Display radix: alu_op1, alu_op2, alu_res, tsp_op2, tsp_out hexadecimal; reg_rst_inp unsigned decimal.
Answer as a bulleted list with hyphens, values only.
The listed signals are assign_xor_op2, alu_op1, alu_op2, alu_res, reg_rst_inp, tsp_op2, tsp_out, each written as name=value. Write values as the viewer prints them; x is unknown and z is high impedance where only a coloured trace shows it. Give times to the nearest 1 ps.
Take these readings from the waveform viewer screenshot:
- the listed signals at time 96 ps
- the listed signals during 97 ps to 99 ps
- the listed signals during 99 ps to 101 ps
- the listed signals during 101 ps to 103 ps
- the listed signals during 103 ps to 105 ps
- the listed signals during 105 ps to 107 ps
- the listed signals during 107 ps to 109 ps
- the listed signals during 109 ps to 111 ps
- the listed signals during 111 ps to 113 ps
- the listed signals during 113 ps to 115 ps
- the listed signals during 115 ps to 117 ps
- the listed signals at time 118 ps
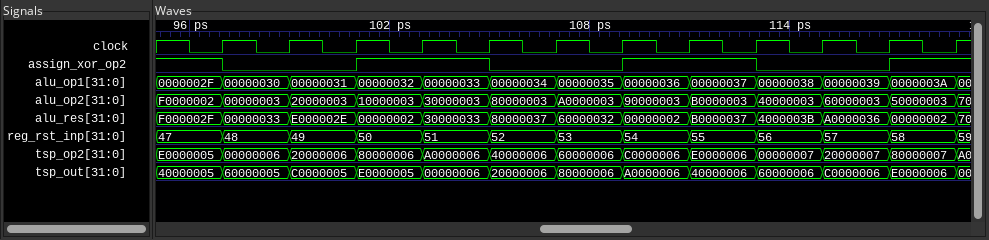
- assign_xor_op2=1, alu_op1=0000002F, alu_op2=F0000002, alu_res=F000002F, reg_rst_inp=47, tsp_op2=E0000005, tsp_out=40000005
- assign_xor_op2=0, alu_op1=00000030, alu_op2=00000003, alu_res=00000033, reg_rst_inp=48, tsp_op2=00000006, tsp_out=60000005
- assign_xor_op2=0, alu_op1=00000031, alu_op2=20000003, alu_res=E000002E, reg_rst_inp=49, tsp_op2=20000006, tsp_out=C0000005
- assign_xor_op2=1, alu_op1=00000032, alu_op2=10000003, alu_res=00000002, reg_rst_inp=50, tsp_op2=80000006, tsp_out=E0000005
- assign_xor_op2=1, alu_op1=00000033, alu_op2=30000003, alu_res=30000033, reg_rst_inp=51, tsp_op2=A0000006, tsp_out=00000006
- assign_xor_op2=0, alu_op1=00000034, alu_op2=80000003, alu_res=80000037, reg_rst_inp=52, tsp_op2=40000006, tsp_out=20000006
- assign_xor_op2=0, alu_op1=00000035, alu_op2=A0000003, alu_res=60000032, reg_rst_inp=53, tsp_op2=60000006, tsp_out=80000006
- assign_xor_op2=1, alu_op1=00000036, alu_op2=90000003, alu_res=00000002, reg_rst_inp=54, tsp_op2=C0000006, tsp_out=A0000006
- assign_xor_op2=1, alu_op1=00000037, alu_op2=B0000003, alu_res=B0000037, reg_rst_inp=55, tsp_op2=E0000006, tsp_out=40000006
- assign_xor_op2=0, alu_op1=00000038, alu_op2=40000003, alu_res=4000003B, reg_rst_inp=56, tsp_op2=00000007, tsp_out=60000006
- assign_xor_op2=0, alu_op1=00000039, alu_op2=60000003, alu_res=A0000036, reg_rst_inp=57, tsp_op2=20000007, tsp_out=C0000006
- assign_xor_op2=1, alu_op1=0000003A, alu_op2=50000003, alu_res=00000002, reg_rst_inp=58, tsp_op2=80000007, tsp_out=E0000006
